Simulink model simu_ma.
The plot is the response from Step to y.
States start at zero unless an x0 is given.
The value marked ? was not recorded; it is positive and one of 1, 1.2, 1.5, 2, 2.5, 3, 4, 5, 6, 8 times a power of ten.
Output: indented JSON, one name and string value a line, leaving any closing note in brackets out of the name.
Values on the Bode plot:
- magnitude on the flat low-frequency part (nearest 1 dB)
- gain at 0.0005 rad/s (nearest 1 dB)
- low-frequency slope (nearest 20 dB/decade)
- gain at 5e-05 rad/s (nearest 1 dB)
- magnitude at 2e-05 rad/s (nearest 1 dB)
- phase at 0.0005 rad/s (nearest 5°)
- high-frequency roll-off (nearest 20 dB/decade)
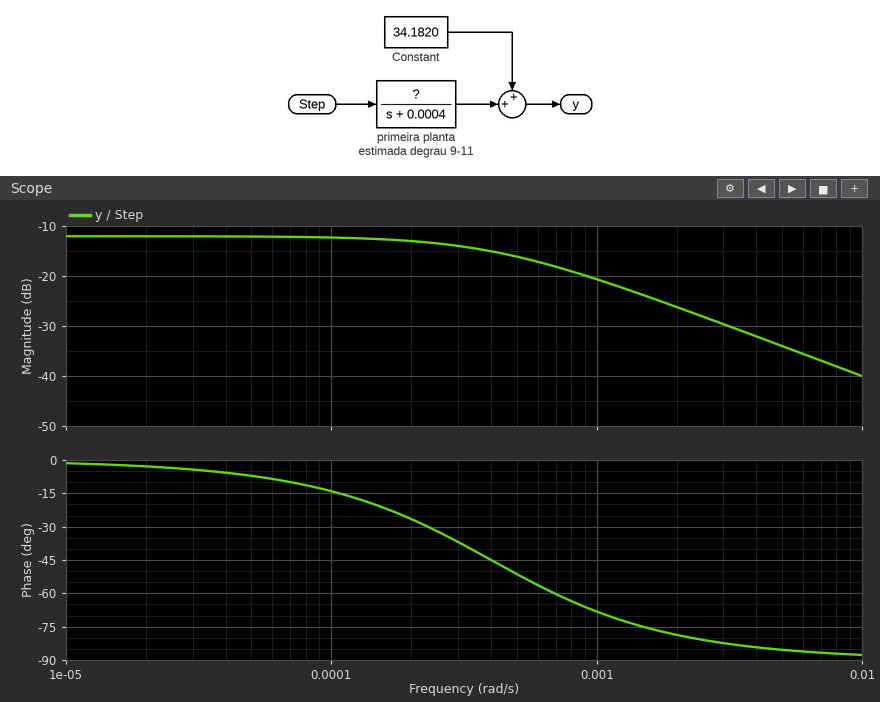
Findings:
{
  "magnitude on the flat low-frequency part": "-12 dB",
  "gain at 0.0005 rad/s": "-16 dB",
  "low-frequency slope": "0 dB/decade",
  "gain at 5e-05 rad/s": "-12 dB",
  "magnitude at 2e-05 rad/s": "-12 dB",
  "phase at 0.0005 rad/s": "-50°",
  "high-frequency roll-off": "-20 dB/decade"
}
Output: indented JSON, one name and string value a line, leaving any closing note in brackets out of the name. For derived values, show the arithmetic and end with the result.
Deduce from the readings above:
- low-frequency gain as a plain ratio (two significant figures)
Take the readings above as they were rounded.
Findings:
{
  "low-frequency gain as a plain ratio": "10^(-12 / 20) = 0.25"
}
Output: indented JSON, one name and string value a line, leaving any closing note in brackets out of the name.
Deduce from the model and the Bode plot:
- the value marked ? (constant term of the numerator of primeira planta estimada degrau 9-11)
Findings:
{
  "the value marked ?": "0.0001"
}
